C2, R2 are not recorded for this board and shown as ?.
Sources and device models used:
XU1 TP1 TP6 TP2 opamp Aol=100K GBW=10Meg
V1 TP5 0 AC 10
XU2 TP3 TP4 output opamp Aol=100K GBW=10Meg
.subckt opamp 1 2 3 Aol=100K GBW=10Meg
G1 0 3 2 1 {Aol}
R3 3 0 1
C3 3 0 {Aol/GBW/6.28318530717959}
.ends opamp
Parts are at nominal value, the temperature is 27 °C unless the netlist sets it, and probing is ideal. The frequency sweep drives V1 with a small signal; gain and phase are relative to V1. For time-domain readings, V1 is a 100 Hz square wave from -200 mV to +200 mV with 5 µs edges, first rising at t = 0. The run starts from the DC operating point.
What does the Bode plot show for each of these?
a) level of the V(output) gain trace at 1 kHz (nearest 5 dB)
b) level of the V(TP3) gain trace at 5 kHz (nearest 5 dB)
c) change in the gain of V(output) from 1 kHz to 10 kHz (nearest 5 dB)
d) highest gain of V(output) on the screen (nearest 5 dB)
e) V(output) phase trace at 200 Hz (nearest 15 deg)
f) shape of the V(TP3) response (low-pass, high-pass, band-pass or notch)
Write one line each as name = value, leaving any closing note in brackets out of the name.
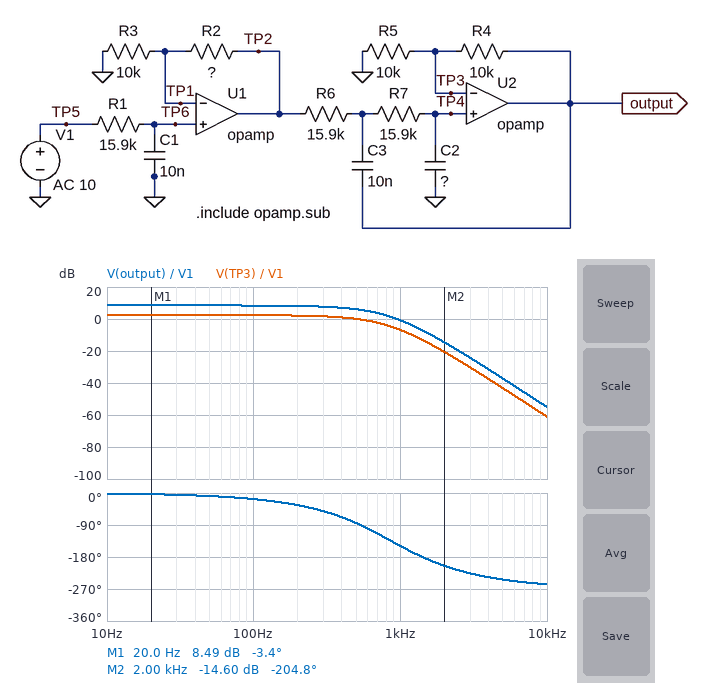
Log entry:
level of the V(output) gain trace at 1 kHz = 0 dB
level of the V(TP3) gain trace at 5 kHz = -45 dB
change in the gain of V(output) from 1 kHz to 10 kHz = -55 dB
highest gain of V(output) on the screen = 10 dB
V(output) phase trace at 200 Hz = -30 deg
shape of the V(TP3) response = low-pass
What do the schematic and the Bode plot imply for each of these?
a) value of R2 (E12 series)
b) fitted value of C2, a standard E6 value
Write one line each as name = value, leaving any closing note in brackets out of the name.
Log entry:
value of R2 = 3.3 kΩ
fitted value of C2, a standard E6 value = 15 nF
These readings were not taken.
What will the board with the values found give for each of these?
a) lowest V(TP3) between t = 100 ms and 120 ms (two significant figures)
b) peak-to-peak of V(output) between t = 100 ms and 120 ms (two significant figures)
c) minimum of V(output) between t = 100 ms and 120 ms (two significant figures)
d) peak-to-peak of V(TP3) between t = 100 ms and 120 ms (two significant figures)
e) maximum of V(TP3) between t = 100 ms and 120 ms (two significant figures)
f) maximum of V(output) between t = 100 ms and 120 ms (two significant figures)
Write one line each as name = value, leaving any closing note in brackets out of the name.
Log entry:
lowest V(TP3) between t = 100 ms and 120 ms = -270 mV
peak-to-peak of V(output) between t = 100 ms and 120 ms = 1.1 V
minimum of V(output) between t = 100 ms and 120 ms = -540 mV
peak-to-peak of V(TP3) between t = 100 ms and 120 ms = 540 mV
maximum of V(TP3) between t = 100 ms and 120 ms = 270 mV
maximum of V(output) between t = 100 ms and 120 ms = 540 mV
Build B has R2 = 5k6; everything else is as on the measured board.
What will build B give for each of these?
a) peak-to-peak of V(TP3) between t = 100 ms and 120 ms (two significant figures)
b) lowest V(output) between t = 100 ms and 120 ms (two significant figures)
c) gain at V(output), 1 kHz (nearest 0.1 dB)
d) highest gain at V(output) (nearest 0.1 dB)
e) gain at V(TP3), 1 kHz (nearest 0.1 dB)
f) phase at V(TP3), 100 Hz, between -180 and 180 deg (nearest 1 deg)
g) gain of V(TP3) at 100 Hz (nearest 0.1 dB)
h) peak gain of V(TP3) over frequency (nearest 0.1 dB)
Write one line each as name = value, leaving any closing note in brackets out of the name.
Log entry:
peak-to-peak of V(TP3) between t = 100 ms and 120 ms = 630 mV
lowest V(output) between t = 100 ms and 120 ms = -630 mV
gain at V(output), 1 kHz = 0.6 dB
highest gain at V(output) = 9.9 dB
gain at V(TP3), 1 kHz = -5.4 dB
phase at V(TP3), 100 Hz, between -180 and 180 deg = -17 deg
gain of V(TP3) at 100 Hz = 3.8 dB
peak gain of V(TP3) over frequency = 3.9 dB
